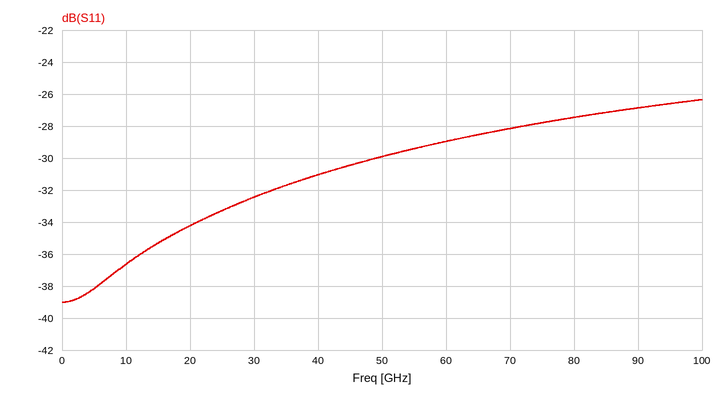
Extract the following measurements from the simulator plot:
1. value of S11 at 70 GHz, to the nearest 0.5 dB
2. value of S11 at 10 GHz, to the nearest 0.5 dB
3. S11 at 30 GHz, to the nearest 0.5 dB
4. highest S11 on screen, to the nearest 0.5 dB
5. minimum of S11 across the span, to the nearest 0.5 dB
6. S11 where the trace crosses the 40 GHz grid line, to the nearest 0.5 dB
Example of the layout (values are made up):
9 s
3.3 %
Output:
-28.0 dB
-36.5 dB
-32.5 dB
-26.5 dB
-39.0 dB
-31.0 dB
